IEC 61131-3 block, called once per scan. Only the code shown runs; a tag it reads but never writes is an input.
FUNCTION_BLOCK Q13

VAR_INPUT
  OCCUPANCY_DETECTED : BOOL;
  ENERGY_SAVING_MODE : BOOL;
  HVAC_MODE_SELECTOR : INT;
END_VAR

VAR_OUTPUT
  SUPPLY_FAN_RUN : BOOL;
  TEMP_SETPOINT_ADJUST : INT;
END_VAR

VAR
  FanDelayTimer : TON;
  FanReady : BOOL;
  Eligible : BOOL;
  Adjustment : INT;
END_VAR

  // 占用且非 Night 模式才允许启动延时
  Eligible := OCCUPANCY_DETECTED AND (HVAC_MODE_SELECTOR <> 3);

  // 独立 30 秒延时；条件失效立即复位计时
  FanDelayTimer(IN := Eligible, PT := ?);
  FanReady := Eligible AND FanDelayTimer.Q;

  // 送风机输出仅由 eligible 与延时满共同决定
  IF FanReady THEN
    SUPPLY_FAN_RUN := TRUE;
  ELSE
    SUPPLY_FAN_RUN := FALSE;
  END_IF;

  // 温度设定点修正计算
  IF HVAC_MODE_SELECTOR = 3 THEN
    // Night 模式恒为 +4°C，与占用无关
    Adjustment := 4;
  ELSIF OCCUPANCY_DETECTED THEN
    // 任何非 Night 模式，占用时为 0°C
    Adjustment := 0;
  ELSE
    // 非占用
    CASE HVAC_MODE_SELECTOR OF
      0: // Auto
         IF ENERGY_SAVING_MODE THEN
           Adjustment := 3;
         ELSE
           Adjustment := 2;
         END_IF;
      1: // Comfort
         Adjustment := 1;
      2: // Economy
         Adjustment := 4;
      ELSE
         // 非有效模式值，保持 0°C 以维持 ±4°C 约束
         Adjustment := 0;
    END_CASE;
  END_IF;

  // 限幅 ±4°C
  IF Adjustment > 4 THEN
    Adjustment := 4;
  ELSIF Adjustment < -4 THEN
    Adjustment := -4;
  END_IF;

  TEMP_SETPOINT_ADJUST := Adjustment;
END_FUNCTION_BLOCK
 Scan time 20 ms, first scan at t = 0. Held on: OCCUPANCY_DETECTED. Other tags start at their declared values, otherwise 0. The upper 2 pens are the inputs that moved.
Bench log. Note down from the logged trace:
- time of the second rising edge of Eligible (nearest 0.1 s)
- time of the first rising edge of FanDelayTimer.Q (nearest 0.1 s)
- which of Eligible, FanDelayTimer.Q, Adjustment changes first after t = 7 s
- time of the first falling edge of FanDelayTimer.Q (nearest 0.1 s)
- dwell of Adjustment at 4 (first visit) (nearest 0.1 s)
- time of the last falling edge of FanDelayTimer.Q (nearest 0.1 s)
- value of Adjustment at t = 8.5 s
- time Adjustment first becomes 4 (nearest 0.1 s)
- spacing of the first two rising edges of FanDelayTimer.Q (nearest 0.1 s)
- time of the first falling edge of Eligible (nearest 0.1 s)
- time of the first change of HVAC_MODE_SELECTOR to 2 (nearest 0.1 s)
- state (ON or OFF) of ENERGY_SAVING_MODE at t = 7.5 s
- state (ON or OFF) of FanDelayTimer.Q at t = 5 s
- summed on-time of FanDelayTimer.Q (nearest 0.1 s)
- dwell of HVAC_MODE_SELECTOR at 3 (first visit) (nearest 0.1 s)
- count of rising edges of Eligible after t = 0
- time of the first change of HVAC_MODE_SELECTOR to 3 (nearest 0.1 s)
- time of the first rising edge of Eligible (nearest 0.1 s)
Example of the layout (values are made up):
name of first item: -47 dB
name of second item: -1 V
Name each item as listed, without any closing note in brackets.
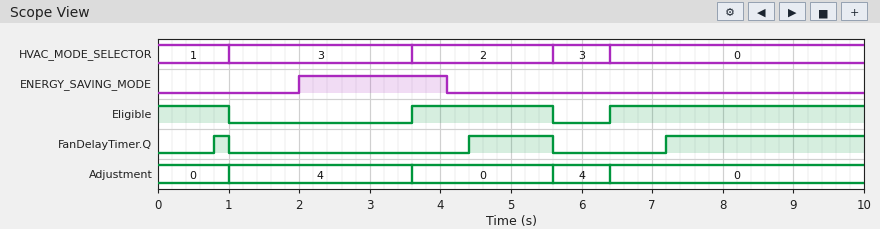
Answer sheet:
time of the second rising edge of Eligible: 6.4 s
time of the first rising edge of FanDelayTimer.Q: 0.8 s
which of Eligible, FanDelayTimer.Q, Adjustment changes first after t = 7 s: FanDelayTimer.Q
time of the first falling edge of FanDelayTimer.Q: 1.0 s
dwell of Adjustment at 4 (first visit): 2.6 s
time of the last falling edge of FanDelayTimer.Q: 5.6 s
value of Adjustment at t = 8.5 s: 0
time Adjustment first becomes 4: 1.0 s
spacing of the first two rising edges of FanDelayTimer.Q: 3.6 s
time of the first falling edge of Eligible: 1.0 s
time of the first change of HVAC_MODE_SELECTOR to 2: 3.6 s
state (ON or OFF) of ENERGY_SAVING_MODE at t = 7.5 s: OFF
state (ON or OFF) of FanDelayTimer.Q at t = 5 s: ON
summed on-time of FanDelayTimer.Q: 4.2 s
dwell of HVAC_MODE_SELECTOR at 3 (first visit): 2.6 s
count of rising edges of Eligible after t = 0: 2
time of the first change of HVAC_MODE_SELECTOR to 3: 1.0 s
time of the first rising edge of Eligible: 3.6 s
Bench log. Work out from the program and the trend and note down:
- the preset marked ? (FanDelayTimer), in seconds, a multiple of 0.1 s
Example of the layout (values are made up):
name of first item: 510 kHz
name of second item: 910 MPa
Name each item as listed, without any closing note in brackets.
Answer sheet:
the preset marked ? (FanDelayTimer), in seconds, a multiple of 0.1 s: 0.8 s
